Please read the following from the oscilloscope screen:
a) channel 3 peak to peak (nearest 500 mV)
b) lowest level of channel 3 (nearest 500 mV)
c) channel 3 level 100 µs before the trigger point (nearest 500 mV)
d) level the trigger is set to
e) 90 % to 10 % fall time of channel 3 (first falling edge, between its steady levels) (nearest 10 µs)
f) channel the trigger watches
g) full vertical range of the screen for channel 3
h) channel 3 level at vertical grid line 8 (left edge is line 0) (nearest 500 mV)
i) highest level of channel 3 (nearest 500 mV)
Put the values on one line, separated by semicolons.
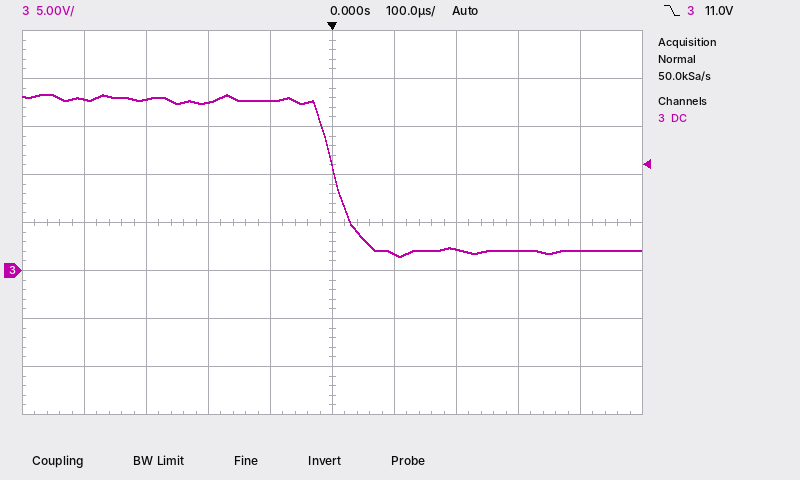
17.0 V; 1.5 V; 17.5 V; 11.0 V; 70 µs; channel 3; 40 V; 2.0 V; 18.5 V
